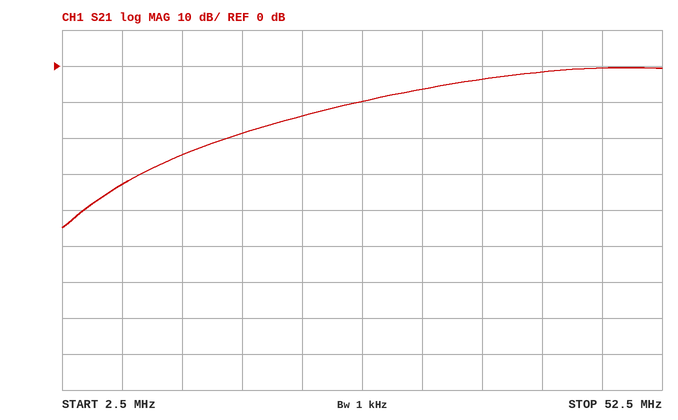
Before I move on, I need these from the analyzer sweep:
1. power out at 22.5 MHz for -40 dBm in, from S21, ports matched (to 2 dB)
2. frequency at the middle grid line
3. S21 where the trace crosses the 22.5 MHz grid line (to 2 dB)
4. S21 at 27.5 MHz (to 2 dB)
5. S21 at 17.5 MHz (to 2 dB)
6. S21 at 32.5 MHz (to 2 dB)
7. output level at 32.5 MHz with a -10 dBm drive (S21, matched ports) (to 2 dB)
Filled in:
-54 dBm
27.5 MHz
-14 dB
-10 dB
-18 dB
-6 dB
-16 dBm
